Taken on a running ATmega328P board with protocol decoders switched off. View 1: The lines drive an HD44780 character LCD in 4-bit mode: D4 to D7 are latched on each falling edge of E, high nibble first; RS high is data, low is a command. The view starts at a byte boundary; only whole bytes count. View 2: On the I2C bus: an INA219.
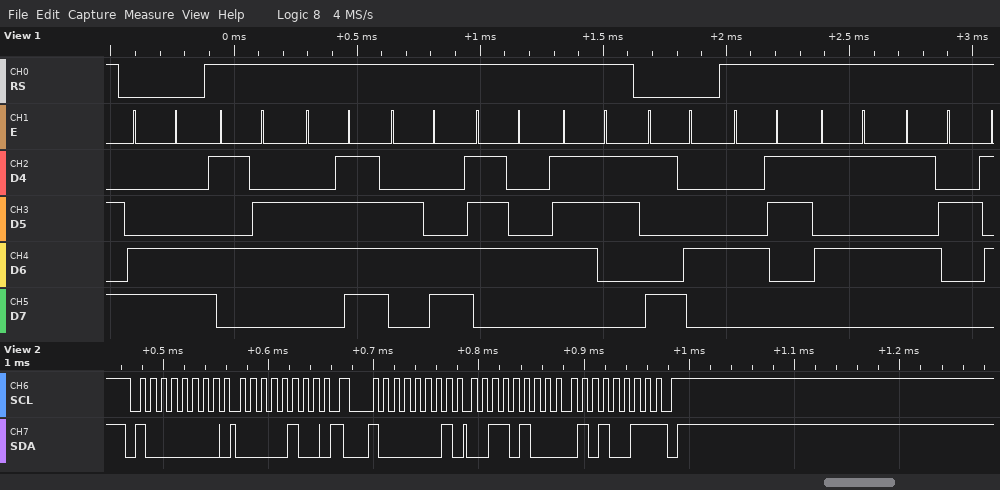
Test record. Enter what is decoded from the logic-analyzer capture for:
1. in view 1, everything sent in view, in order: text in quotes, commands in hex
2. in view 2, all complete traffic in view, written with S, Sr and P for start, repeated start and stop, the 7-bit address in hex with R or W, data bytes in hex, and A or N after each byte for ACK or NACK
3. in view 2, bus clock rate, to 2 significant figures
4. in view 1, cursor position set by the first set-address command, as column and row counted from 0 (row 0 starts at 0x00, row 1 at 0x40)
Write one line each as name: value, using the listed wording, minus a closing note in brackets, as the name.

in view 1, everything sent in view, in order: text in quotes, commands in hex: 0xCC "Volts" 0x94 "CUR"
in view 2, all complete traffic in view, written with S, Sr and P for start, repeated start and stop, the 7-bit address in hex with R or W, data bytes in hex, and A or N after each byte for ACK or NACK: S 40W A 04 A Sr 40R A 34 A 53 N P
in view 2, bus clock rate, to 2 significant figures: 100 kHz
in view 1, cursor position set by the first set-address command, as column and row counted from 0: column 12, row 1
